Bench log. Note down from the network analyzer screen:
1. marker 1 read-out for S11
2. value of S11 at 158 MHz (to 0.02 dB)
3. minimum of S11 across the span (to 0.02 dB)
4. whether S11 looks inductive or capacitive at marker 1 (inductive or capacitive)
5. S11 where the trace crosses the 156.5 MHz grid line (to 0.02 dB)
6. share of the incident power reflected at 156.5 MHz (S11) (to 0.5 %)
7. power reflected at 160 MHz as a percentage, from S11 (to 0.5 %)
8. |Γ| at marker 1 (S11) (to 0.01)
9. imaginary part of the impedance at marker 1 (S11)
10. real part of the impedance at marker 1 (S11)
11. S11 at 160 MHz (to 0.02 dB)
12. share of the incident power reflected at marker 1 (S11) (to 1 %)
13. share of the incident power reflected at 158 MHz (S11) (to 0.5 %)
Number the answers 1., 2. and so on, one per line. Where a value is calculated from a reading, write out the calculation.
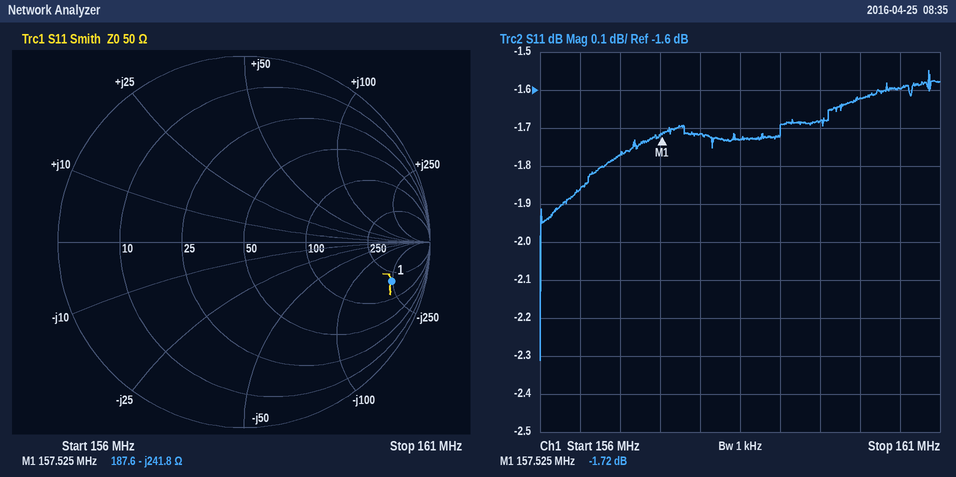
1. -1.72 dB
2. -1.72 dB
3. -2.32 dB
4. capacitive
5. -1.86 dB
6. 10^(-1.86/10) ≈ 65.2 %, so 65.0 % to the nearest 0.5 %
7. 10^(-1.62/10) ≈ 68.9 %, so 69.0 % to the nearest 0.5 %
8. 0.82
9. -241.8 Ω
10. 187.6 Ω
11. -1.62 dB
12. 10^(-1.72/10) ≈ 67 %
13. 10^(-1.72/10) ≈ 67.3 %, so 67.5 % to the nearest 0.5 %
